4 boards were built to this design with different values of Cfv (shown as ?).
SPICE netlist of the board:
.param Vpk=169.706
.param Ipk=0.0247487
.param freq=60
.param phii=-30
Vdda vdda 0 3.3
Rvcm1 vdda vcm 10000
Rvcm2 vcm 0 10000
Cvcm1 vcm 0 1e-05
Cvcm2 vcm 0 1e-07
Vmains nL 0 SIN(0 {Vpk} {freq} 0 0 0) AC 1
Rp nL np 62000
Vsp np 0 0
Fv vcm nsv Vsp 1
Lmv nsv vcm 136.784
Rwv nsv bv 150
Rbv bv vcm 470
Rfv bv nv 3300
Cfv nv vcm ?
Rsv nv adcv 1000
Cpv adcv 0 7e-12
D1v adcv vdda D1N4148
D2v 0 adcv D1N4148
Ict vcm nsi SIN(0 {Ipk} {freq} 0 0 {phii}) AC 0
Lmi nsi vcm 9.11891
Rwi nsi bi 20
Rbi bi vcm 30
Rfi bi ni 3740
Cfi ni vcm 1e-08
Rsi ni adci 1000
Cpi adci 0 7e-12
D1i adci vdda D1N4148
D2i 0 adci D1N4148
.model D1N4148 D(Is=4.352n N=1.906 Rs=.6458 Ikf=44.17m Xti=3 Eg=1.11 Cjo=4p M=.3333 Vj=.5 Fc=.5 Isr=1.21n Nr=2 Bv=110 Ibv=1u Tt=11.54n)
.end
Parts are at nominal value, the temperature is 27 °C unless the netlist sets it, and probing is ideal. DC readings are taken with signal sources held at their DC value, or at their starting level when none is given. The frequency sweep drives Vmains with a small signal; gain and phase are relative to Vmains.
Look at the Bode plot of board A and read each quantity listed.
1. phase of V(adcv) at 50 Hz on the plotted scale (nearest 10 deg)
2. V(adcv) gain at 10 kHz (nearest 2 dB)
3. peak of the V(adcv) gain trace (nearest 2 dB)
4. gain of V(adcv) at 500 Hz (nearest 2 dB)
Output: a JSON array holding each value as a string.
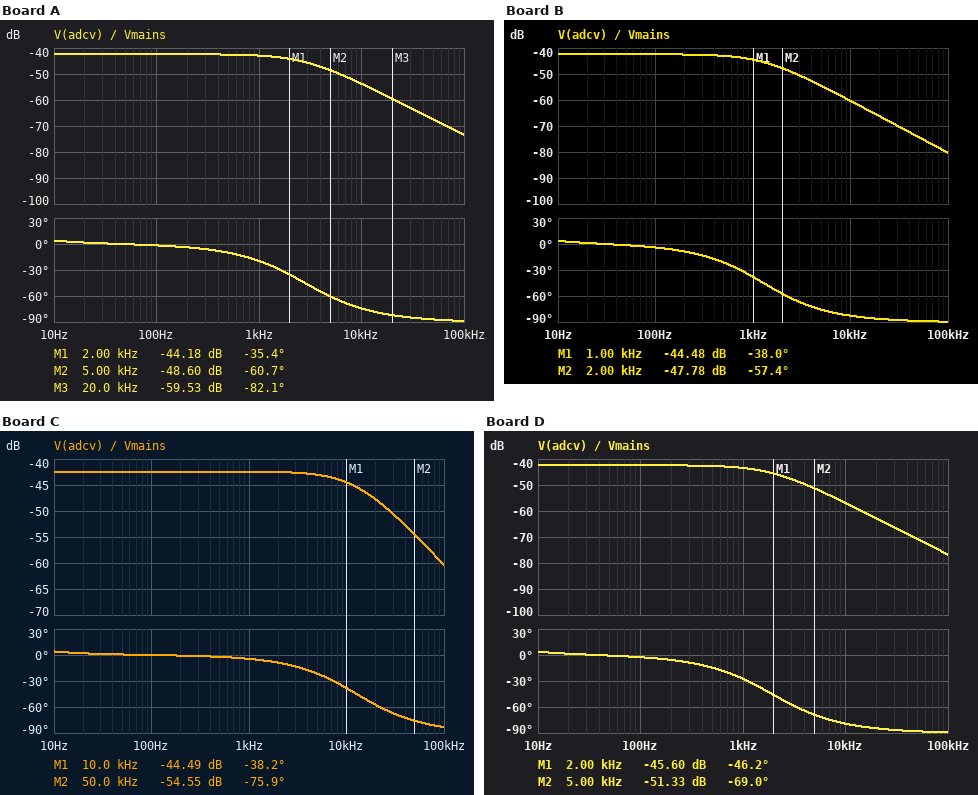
["0 deg", "-54 dB", "-42 dB", "-42 dB"]
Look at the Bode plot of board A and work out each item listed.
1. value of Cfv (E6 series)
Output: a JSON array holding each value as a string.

["15 nF"]
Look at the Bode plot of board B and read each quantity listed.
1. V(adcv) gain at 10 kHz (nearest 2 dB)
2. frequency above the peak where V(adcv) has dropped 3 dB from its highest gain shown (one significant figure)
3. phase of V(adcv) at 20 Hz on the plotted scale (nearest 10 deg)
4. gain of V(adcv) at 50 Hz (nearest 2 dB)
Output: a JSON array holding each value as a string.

["-60 dB", "1 kHz", "0 deg", "-42 dB"]
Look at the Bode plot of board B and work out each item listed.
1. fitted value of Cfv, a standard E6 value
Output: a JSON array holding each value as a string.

["33 nF"]
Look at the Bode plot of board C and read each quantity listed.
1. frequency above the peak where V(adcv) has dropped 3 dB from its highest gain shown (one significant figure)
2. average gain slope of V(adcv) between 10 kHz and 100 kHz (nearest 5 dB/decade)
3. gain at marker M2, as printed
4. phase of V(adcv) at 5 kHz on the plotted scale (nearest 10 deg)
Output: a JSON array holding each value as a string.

["10 kHz", "-15 dB/decade", "-54.55 dB", "-20 deg"]
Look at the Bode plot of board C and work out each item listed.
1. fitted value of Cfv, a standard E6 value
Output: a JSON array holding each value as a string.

["3.3 nF"]
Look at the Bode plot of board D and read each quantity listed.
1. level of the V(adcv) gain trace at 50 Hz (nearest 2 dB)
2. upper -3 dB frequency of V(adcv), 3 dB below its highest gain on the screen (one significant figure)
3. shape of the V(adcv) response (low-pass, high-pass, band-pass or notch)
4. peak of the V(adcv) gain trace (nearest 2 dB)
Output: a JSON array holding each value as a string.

["-42 dB", "2 kHz", "low-pass", "-42 dB"]
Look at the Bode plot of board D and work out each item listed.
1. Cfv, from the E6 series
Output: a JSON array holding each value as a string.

["22 nF"]
